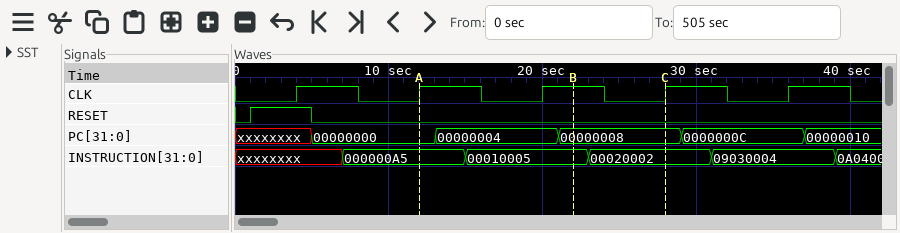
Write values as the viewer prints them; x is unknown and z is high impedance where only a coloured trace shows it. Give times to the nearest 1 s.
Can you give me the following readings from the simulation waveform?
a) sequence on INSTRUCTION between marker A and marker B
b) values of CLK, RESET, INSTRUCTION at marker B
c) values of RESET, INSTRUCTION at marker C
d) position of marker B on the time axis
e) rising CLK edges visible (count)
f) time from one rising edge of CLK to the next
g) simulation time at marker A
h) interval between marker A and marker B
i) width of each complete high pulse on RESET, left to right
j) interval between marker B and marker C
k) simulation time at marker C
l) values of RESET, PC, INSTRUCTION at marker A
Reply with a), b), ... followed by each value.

a) 000000A5, 00010005
b) CLK=1, RESET=0, INSTRUCTION=00010005
c) RESET=0, INSTRUCTION=00020002
d) 22 s
e) 5
f) 8 s
g) 12 s
h) 10 s
i) 4 s
j) 6 s
k) 28 s
l) RESET=0, PC=00000000, INSTRUCTION=000000A5
